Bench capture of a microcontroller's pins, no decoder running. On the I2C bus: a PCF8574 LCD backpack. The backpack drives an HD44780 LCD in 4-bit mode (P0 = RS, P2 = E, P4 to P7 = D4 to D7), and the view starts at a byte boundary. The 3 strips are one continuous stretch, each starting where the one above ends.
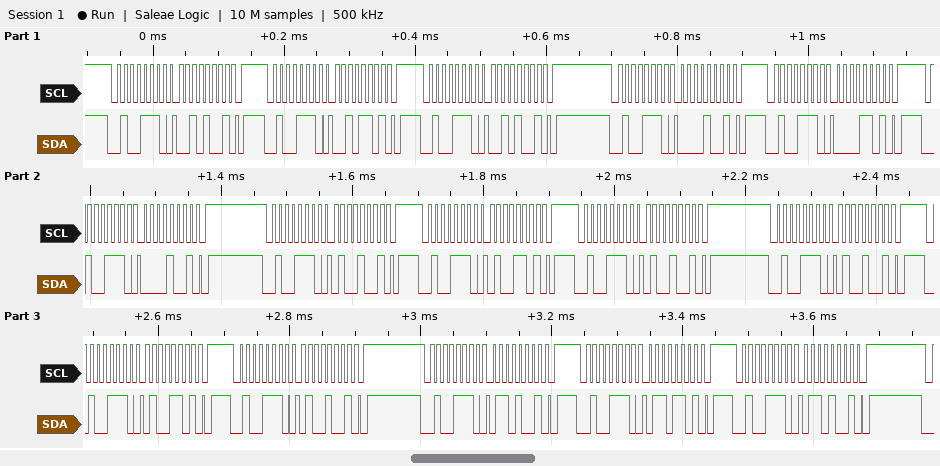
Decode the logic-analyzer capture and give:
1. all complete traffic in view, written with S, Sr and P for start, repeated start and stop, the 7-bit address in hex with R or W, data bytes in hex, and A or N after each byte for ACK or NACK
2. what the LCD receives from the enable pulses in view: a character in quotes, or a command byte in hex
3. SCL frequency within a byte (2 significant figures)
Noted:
S 27W A 29 A P S 27W A 2D A P S 27W A 29 A P S 27W A 09 A P S 27W A 0D A P S 27W A 09 A P S 27W A 49 A P S 27W A 4D A P S 27W A 49 A P S 27W A 49 A P S 27W A 4D A P S 27W A 49 A P S 27W A 69 A P S 27W A 6D A P S 27W A 69 A P
' ' 'D'
100 kHz
